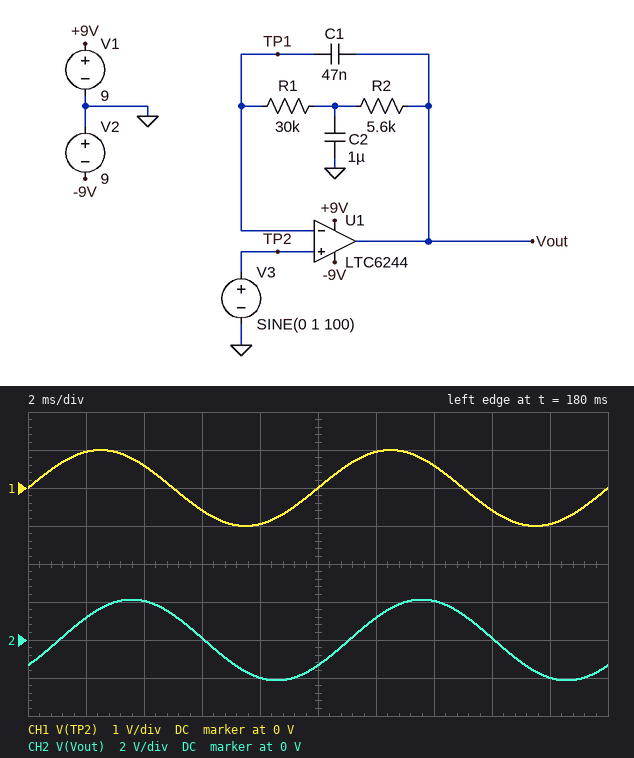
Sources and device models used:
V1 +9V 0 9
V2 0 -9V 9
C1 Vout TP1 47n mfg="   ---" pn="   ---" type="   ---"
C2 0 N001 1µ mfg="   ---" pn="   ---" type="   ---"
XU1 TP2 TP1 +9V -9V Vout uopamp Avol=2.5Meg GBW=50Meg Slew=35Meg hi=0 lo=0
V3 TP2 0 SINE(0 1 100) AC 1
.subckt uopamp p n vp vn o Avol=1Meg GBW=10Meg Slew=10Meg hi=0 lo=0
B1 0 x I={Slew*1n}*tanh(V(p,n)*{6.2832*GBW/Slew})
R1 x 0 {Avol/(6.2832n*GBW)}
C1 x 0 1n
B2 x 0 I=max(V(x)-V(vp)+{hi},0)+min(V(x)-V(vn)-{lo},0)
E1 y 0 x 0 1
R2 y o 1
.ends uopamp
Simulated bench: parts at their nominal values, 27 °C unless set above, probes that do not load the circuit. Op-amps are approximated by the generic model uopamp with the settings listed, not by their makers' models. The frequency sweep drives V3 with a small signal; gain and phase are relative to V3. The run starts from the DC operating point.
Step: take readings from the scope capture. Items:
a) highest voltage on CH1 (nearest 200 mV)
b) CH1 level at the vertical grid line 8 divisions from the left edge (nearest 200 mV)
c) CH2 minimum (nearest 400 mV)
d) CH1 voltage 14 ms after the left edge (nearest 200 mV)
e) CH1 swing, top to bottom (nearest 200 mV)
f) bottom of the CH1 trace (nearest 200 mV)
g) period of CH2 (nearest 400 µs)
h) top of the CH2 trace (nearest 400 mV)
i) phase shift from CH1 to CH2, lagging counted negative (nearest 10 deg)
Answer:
1.0 V
-600 mV
-2.0 V
600 mV
2.0 V
-1.0 V
10.0 ms
2.0 V
-40 deg
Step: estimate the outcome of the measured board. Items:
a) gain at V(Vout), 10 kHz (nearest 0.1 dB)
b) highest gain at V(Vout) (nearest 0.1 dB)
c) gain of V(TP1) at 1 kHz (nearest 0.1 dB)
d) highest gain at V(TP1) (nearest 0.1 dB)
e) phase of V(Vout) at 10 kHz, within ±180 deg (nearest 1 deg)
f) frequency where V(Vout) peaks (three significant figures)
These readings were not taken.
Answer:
0 dB
12.8 dB
0 dB
0 dB
-1 deg
56.6 Hz
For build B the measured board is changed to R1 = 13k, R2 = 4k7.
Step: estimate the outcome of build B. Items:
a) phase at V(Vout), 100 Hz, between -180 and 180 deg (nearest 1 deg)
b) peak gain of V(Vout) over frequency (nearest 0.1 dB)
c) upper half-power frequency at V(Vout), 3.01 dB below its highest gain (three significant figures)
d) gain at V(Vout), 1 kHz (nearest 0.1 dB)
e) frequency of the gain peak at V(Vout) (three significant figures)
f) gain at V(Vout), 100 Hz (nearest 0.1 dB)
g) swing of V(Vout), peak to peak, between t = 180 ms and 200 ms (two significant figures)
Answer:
-12 deg
16.5 dB
120 Hz
0.4 dB
93.9 Hz
16.2 dB
13 V
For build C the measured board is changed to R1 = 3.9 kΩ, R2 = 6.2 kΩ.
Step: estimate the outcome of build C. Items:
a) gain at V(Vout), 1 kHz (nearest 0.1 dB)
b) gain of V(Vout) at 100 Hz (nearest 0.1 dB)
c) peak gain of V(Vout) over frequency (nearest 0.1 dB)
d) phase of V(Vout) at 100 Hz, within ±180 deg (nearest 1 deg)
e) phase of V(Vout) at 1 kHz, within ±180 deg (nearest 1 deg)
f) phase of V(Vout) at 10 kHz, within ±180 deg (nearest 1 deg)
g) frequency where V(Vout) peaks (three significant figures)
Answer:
2.8 dB
16.6 dB
23.0 dB
54 deg
-40 deg
-5 deg
149 Hz
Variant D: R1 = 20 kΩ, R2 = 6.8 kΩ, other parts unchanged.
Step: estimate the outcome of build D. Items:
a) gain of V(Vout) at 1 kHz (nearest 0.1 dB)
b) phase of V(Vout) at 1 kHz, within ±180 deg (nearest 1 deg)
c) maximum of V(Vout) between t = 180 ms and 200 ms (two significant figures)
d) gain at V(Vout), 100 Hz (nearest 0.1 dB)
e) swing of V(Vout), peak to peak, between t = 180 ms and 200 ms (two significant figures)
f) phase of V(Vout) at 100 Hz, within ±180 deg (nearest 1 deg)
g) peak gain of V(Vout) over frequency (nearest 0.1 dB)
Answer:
0.2 dB
-10 deg
3.1 V
9.8 dB
6.2 V
-46 deg
16.1 dB
